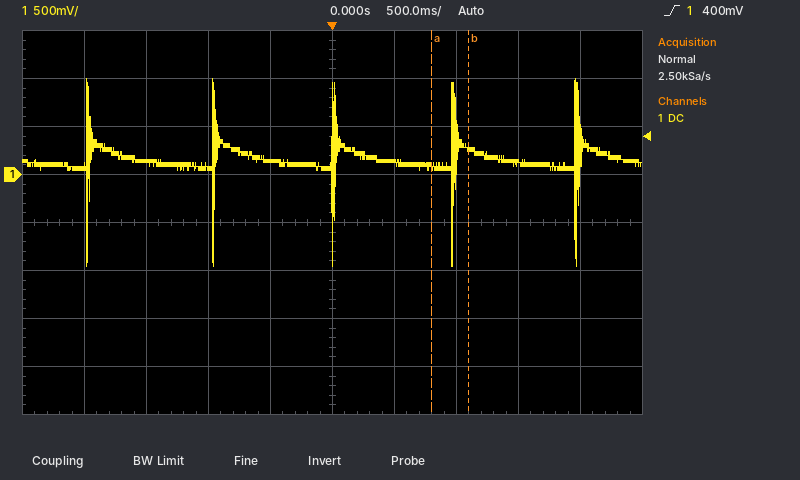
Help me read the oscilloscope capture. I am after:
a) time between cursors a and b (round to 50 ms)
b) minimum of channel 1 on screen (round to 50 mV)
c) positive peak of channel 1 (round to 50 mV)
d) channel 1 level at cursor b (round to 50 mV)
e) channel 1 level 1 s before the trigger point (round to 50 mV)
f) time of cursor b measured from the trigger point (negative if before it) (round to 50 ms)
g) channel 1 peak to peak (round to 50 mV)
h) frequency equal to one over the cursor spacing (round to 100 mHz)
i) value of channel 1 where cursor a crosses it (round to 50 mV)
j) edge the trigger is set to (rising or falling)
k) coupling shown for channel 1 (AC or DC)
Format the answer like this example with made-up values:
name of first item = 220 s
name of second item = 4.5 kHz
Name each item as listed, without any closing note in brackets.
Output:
time between cursors a and b = 300 ms
minimum of channel 1 on screen = -950 mV
positive peak of channel 1 = 1.00 V
channel 1 level at cursor b = 300 mV
channel 1 level 1 s before the trigger point = 100 mV
time of cursor b measured from the trigger point (negative if before it) = +1.10 s
channel 1 peak to peak = 1.95 V
frequency equal to one over the cursor spacing = 3.3 Hz
value of channel 1 where cursor a crosses it = 100 mV
edge the trigger is set to = rising
coupling shown for channel 1 = DC
